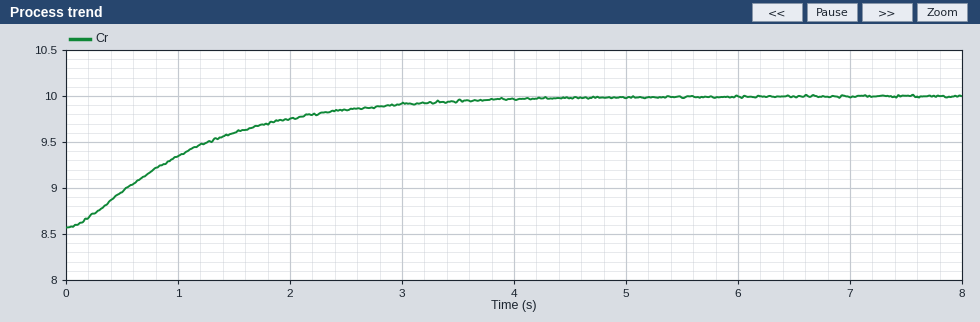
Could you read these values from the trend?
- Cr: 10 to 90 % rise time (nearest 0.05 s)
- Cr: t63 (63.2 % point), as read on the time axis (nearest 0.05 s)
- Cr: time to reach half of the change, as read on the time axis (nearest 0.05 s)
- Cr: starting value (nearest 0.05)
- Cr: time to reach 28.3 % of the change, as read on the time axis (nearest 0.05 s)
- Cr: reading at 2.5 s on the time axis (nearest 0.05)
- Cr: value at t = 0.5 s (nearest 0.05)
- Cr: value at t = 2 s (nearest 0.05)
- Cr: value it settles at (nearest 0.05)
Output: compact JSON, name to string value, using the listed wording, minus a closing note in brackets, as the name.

{"Cr: 10 to 90 % rise time": "2.30 s", "Cr: t63 (63.2 % point), as read on the time axis": "1.20 s", "Cr: time to reach half of the change, as read on the time axis": "0.90 s", "Cr: starting value": "8.55", "Cr: time to reach 28.3 % of the change, as read on the time axis": "0.50 s", "Cr: reading at 2.5 s on the time axis": "9.85", "Cr: value at t = 0.5 s": "8.95", "Cr: value at t = 2 s": "9.75", "Cr: value it settles at": "10.00"}
